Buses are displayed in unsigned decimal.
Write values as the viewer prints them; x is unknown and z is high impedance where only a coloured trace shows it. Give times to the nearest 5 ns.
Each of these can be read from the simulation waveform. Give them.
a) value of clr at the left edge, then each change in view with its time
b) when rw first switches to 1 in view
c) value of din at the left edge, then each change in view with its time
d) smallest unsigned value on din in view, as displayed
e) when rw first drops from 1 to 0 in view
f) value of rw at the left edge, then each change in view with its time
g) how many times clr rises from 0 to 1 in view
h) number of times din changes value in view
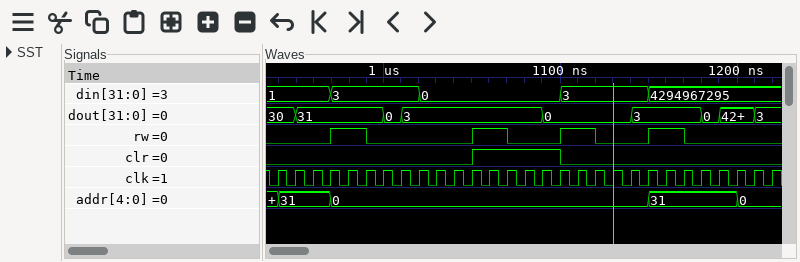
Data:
0, 1 at 1050 ns, 0 at 1100 ns
970 ns
1, 3 at 970 ns, 0 at 1020 ns, 3 at 1100 ns, 4294967295 at 1150 ns
0
990 ns
0, 1 at 970 ns, 0 at 990 ns, 1 at 1050 ns, 0 at 1070 ns, 1 at 1100 ns, 0 at 1120 ns, 1 at 1150 ns, 0 at 1170 ns
1
4
